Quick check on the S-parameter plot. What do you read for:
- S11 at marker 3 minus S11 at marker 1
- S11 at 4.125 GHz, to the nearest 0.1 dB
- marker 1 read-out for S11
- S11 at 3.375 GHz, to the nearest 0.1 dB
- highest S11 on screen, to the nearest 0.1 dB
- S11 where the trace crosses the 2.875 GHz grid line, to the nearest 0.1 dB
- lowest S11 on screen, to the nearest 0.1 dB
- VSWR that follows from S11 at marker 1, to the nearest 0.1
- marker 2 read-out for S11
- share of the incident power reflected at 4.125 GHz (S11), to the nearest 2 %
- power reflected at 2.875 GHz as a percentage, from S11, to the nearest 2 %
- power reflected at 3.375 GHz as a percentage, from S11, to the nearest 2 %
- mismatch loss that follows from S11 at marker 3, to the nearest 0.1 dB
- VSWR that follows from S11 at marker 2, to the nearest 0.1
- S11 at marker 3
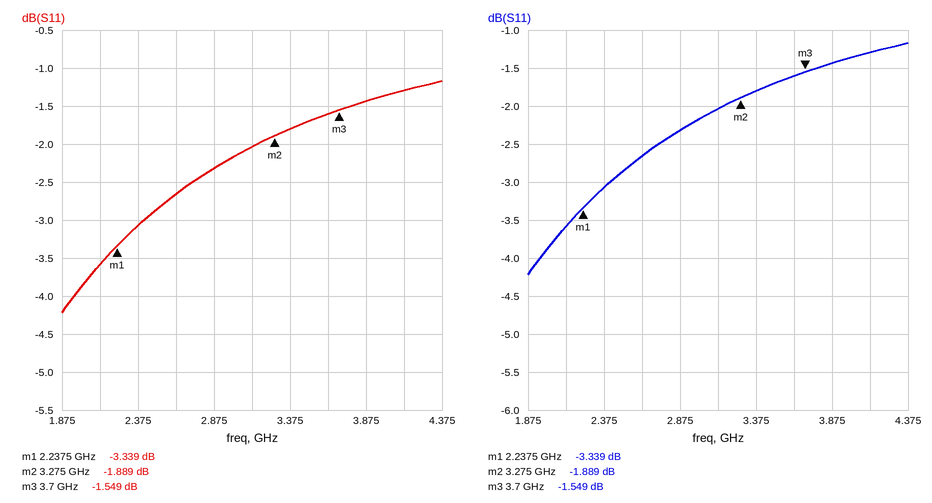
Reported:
1.790 dB
-1.3 dB
-3.339 dB
-1.8 dB
-1.2 dB
-2.3 dB
-4.2 dB
5.3
-1.889 dB
74 %
58 %
66 %
5.2 dB
9.2
-1.549 dB
